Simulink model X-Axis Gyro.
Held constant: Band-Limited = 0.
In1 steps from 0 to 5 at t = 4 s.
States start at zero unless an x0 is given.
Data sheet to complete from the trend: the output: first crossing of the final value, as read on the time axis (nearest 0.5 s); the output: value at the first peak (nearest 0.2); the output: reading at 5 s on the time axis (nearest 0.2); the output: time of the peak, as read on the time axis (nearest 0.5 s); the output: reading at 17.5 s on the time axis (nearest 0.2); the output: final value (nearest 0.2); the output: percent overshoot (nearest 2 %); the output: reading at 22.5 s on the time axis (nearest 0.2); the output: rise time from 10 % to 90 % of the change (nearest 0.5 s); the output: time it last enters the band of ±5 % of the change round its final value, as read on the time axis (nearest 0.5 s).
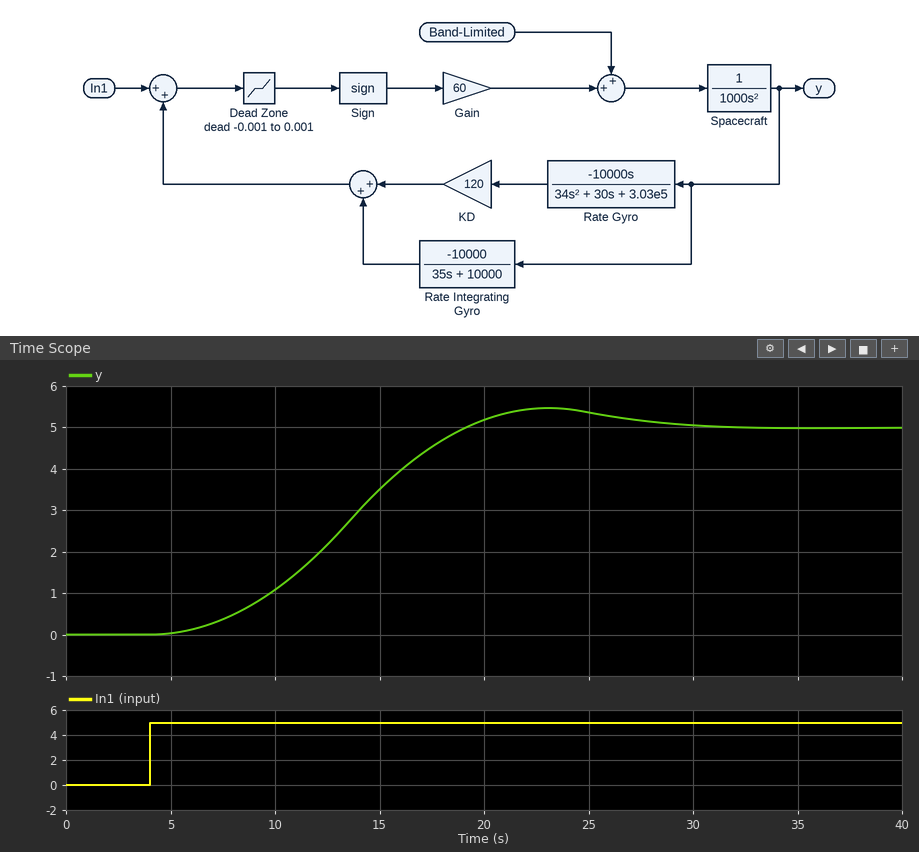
19.0 s
5.4
0.0
23.0 s
4.6
5.0
10 %
5.4
9.5 s
26.5 s
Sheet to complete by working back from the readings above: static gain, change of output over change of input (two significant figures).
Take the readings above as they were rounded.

1.0
